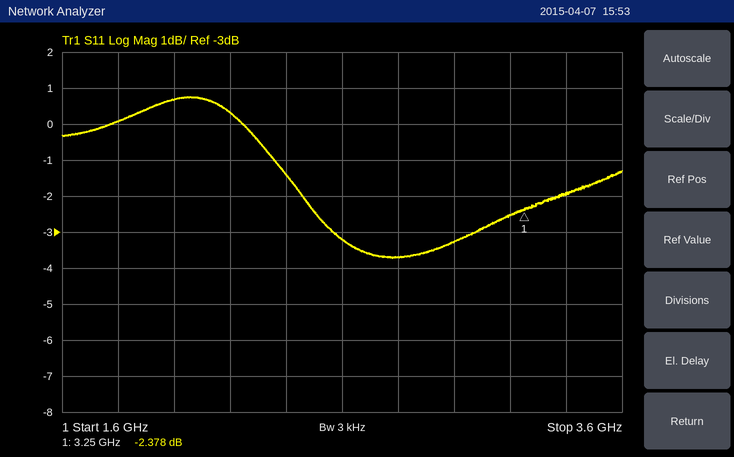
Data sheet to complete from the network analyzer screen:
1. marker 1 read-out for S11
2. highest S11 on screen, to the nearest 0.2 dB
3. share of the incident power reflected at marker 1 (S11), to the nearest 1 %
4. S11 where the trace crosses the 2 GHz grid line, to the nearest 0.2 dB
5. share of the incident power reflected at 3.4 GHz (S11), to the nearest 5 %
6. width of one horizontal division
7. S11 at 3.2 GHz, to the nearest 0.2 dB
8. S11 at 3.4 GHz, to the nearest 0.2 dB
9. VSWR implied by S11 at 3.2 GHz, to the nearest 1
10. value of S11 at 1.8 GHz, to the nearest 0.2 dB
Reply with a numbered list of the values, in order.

1. -2.378 dB
2. 0.8 dB
3. 58 %
4. 0.6 dB
5. 65 %
6. 200 MHz
7. -2.6 dB
8. -2.0 dB
9. 7
10. 0.0 dB
